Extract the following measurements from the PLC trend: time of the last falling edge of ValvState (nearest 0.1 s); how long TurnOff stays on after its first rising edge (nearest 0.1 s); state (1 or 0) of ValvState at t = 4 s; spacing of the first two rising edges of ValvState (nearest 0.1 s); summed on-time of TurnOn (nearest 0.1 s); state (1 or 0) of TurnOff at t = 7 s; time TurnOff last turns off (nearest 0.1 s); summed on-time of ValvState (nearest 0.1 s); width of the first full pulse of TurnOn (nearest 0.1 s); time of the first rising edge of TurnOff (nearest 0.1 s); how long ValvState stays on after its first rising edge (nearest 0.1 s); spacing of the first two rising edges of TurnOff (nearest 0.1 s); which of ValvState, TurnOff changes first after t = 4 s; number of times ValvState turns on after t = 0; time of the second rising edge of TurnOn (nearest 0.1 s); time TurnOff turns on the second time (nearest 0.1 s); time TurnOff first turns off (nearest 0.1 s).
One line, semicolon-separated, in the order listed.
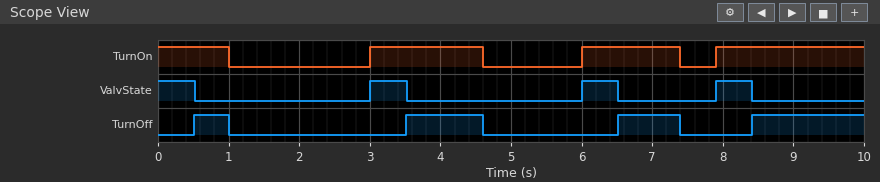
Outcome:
8.4 s; 0.5 s; 0; 3.0 s; 6.1 s; 1; 7.4 s; 2.1 s; 1.6 s; 0.5 s; 0.5 s; 3.0 s; TurnOff; 3; 6.0 s; 3.5 s; 1.0 s
